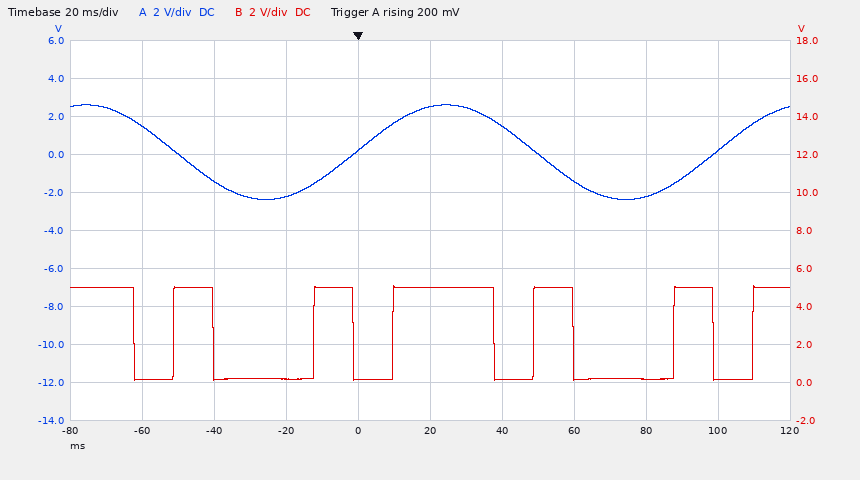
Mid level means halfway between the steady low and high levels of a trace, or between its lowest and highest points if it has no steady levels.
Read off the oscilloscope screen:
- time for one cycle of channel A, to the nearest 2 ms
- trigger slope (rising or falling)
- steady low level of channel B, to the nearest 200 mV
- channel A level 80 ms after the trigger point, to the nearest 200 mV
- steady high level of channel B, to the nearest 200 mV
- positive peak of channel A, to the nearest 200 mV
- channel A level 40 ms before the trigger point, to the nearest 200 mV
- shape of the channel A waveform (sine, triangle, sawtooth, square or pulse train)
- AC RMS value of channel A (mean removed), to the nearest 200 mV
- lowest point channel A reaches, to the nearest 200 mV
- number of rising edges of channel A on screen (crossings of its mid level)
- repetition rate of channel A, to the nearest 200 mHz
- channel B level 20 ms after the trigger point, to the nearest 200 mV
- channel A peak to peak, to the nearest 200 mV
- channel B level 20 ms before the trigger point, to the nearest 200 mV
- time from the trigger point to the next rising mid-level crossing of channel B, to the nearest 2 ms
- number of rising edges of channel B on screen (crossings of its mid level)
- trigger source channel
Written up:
100 ms
rising
200 mV
-2.2 V
5.0 V
2.6 V
-1.4 V
sine
1.8 V
-2.4 V
2
10.0 Hz
5.0 V
5.0 V
200 mV
10 ms
6
channel A
